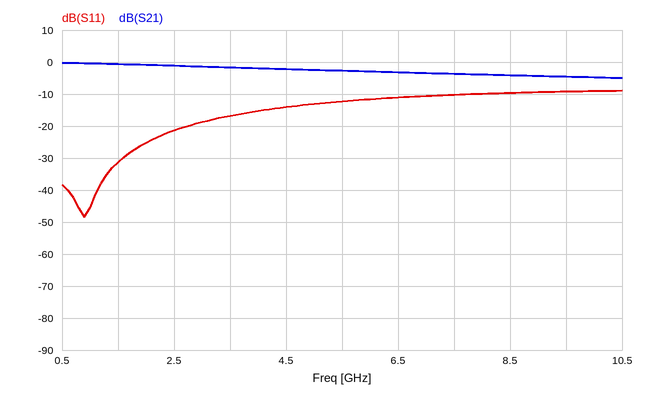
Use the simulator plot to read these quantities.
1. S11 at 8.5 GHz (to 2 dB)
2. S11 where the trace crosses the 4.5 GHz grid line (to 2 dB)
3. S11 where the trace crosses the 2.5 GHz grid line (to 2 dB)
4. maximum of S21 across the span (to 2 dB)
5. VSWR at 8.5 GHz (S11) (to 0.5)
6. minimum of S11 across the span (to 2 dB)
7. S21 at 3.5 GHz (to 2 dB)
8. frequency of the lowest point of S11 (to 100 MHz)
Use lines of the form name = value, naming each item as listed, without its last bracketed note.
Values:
S11 at 8.5 GHz = -10 dB
S11 where the trace crosses the 4.5 GHz grid line = -14 dB
S11 where the trace crosses the 2.5 GHz grid line = -22 dB
maximum of S21 across the span = 0 dB
VSWR at 8.5 GHz (S11) = 2.0
minimum of S11 across the span = -48 dB
S21 at 3.5 GHz = -2 dB
frequency of the lowest point of S11 = 900 MHz
